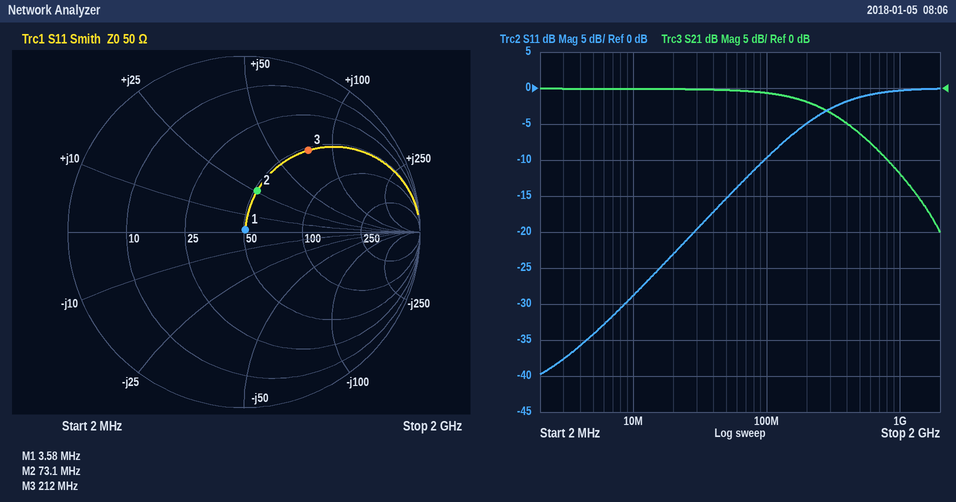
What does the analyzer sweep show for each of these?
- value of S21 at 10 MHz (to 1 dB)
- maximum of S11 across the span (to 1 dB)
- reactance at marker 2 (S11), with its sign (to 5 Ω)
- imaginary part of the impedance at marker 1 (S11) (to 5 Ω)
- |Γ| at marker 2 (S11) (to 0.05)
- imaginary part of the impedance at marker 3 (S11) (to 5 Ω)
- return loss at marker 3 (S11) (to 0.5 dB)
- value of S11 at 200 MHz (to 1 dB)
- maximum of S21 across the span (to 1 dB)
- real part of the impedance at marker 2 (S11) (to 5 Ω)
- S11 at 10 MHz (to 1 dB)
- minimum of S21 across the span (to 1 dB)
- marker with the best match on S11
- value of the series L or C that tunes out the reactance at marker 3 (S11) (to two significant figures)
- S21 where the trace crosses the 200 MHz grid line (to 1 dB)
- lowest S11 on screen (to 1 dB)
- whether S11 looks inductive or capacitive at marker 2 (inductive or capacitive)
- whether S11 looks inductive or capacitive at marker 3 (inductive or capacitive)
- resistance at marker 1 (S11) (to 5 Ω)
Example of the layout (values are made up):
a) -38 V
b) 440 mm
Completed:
a) 0 dB
b) 0 dB
c) +25 Ω
d) 0 Ω
e) 0.25
f) +75 Ω
g) 4.5 dB
h) -5 dB
i) 0 dB
j) 50 Ω
k) -29 dB
l) -20 dB
m) marker 1
n) 10 pF
o) -2 dB
p) -40 dB
q) inductive
r) inductive
s) 50 Ω
